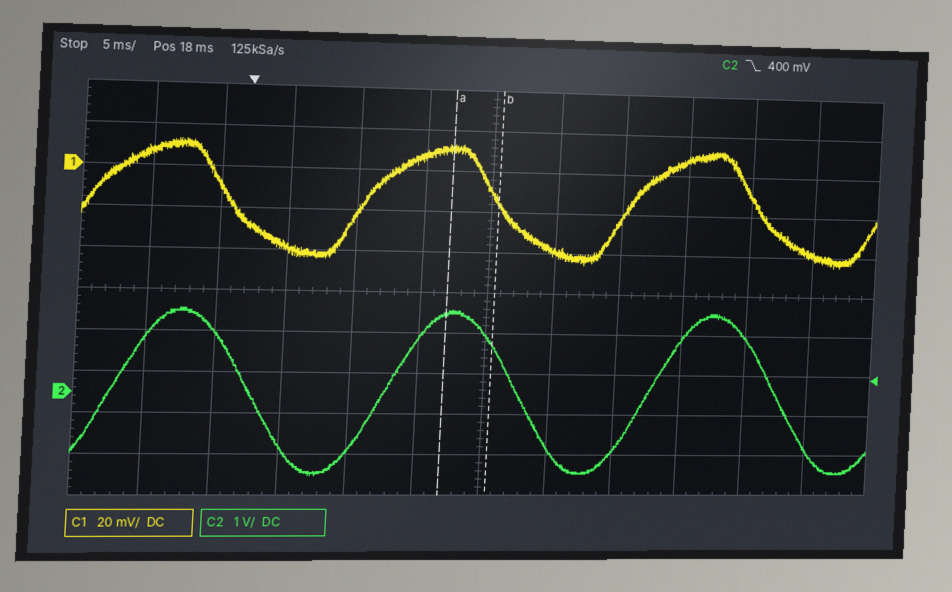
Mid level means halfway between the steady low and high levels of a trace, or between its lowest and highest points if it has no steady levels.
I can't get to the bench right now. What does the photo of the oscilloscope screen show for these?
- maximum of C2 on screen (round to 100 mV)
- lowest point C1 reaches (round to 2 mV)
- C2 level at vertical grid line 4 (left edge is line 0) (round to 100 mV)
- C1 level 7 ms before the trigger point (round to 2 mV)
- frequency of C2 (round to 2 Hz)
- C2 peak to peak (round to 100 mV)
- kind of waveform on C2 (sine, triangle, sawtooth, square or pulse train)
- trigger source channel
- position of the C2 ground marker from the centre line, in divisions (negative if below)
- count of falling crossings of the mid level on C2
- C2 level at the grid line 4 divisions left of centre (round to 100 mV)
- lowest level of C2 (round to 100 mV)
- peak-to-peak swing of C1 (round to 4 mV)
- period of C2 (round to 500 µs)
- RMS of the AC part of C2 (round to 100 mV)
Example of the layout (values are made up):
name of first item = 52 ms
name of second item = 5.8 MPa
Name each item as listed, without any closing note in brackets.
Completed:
maximum of C2 on screen = 2.1 V
lowest point C1 reaches = -44 mV
C2 level at vertical grid line 4 (left edge is line 0) = -1.4 V
C1 level 7 ms before the trigger point = 8 mV
frequency of C2 = 50 Hz
C2 peak to peak = 4.1 V
kind of waveform on C2 = sine
trigger source channel = C2
position of the C2 ground marker from the centre line, in divisions = -2.5 div
count of falling crossings of the mid level on C2 = 3
C2 level at the grid line 4 divisions left of centre = 1.5 V
lowest level of C2 = -2.0 V
peak-to-peak swing of C1 = 56 mV
period of C2 = 20.0 ms
RMS of the AC part of C2 = 1.4 V
